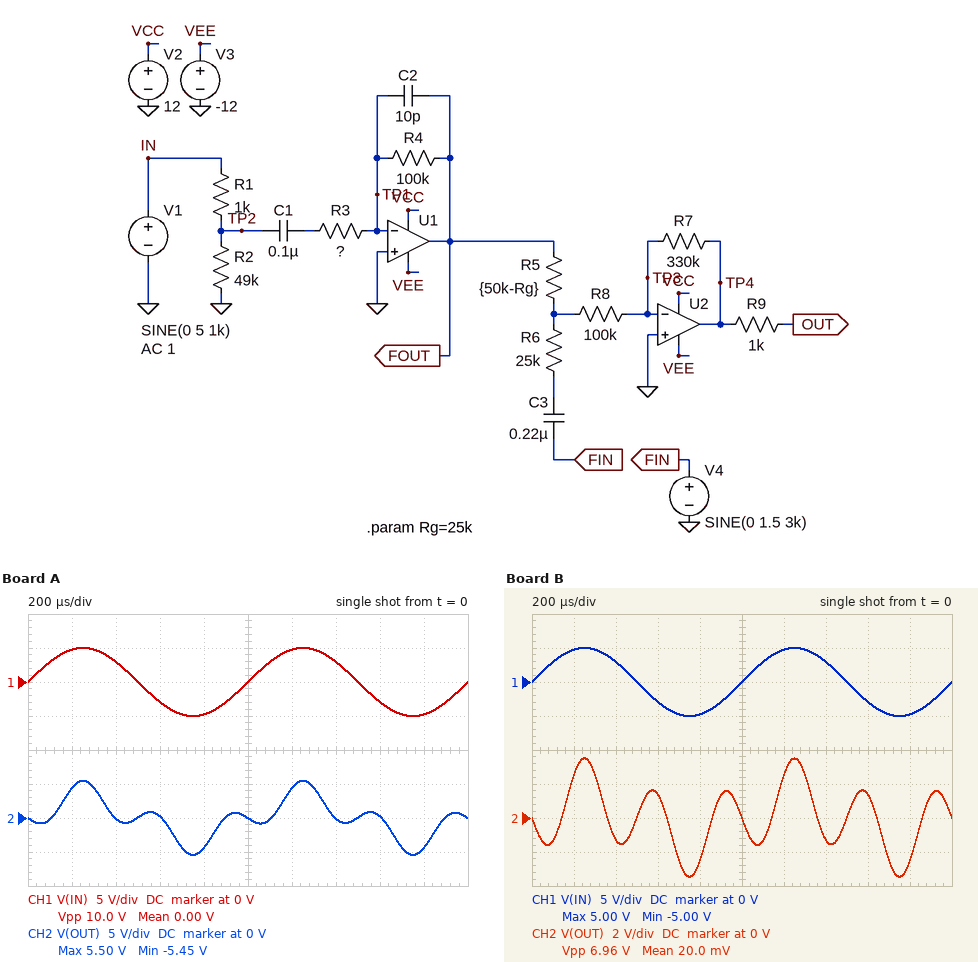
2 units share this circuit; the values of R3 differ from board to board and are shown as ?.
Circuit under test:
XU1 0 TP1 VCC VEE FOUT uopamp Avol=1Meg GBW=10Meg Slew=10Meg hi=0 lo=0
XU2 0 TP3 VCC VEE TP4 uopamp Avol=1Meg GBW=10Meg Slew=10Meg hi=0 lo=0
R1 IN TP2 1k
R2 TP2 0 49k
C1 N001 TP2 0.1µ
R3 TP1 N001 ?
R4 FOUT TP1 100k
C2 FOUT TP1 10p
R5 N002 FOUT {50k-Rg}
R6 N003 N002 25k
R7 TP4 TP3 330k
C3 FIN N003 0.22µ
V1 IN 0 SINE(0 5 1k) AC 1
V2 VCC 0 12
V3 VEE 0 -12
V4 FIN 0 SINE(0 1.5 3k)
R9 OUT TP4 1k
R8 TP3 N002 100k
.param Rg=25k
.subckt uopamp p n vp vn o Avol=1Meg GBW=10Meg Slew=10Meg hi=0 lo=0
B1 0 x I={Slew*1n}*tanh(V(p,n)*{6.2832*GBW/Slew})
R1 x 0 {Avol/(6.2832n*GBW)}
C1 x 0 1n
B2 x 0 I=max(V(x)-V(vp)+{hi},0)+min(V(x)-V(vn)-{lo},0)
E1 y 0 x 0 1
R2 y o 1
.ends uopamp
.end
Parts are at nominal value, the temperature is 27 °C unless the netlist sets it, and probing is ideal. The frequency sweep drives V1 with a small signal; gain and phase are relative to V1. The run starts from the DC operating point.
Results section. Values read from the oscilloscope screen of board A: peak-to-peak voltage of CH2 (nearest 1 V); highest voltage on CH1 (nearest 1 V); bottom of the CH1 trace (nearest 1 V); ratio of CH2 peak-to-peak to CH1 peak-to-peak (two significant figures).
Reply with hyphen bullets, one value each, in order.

- 11 V
- 5 V
- -5 V
- 1.1
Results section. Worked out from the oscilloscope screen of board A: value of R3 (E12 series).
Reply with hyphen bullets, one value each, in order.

- 220 kΩ
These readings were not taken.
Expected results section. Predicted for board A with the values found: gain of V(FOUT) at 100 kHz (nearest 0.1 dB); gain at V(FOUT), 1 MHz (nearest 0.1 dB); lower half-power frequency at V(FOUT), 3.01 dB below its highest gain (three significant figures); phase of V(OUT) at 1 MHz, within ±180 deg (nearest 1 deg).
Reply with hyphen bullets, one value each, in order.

- -8.5 dB
- -23.2 dB
- 7.20 Hz
- -108 deg
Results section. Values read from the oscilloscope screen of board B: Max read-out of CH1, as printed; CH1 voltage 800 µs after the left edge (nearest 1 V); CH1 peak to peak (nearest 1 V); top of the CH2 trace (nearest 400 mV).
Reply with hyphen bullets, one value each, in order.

- 5.00 V
- -5 V
- 10 V
- 3.6 V
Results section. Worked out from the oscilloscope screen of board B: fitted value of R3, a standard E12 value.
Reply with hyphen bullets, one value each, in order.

- 560 kΩ
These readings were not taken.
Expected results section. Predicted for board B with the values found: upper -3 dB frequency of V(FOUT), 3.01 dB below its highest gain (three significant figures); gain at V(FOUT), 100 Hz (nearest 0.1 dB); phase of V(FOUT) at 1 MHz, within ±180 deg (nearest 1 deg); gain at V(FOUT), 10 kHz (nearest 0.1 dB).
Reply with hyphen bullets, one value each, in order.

- 159 kHz
- -15.2 dB
- 93 deg
- -15.2 dB
